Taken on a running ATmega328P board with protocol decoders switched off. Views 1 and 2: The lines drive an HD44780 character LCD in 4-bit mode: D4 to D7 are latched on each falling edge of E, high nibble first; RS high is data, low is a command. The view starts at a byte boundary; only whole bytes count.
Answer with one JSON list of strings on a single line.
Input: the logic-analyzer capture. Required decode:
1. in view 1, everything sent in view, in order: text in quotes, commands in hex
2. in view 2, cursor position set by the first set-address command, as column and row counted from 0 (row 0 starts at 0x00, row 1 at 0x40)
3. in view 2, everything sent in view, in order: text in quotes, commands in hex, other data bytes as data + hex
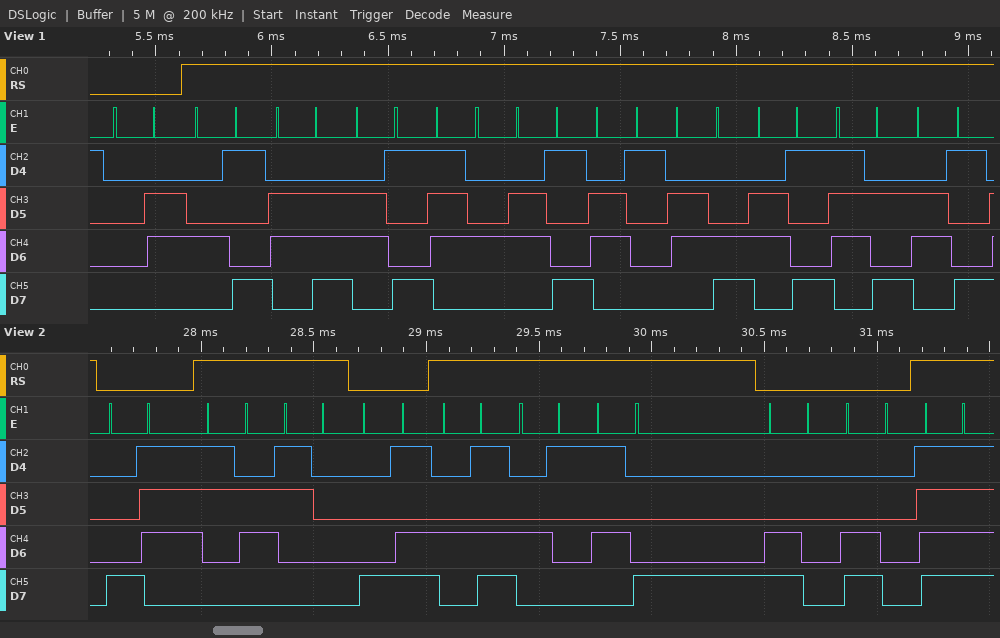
["0x06 \"Initializi\"", "column 7, row 0", "0x87 \"60\" 0x8D \"MAX\" 0xC0 0xC0 data FF"]
